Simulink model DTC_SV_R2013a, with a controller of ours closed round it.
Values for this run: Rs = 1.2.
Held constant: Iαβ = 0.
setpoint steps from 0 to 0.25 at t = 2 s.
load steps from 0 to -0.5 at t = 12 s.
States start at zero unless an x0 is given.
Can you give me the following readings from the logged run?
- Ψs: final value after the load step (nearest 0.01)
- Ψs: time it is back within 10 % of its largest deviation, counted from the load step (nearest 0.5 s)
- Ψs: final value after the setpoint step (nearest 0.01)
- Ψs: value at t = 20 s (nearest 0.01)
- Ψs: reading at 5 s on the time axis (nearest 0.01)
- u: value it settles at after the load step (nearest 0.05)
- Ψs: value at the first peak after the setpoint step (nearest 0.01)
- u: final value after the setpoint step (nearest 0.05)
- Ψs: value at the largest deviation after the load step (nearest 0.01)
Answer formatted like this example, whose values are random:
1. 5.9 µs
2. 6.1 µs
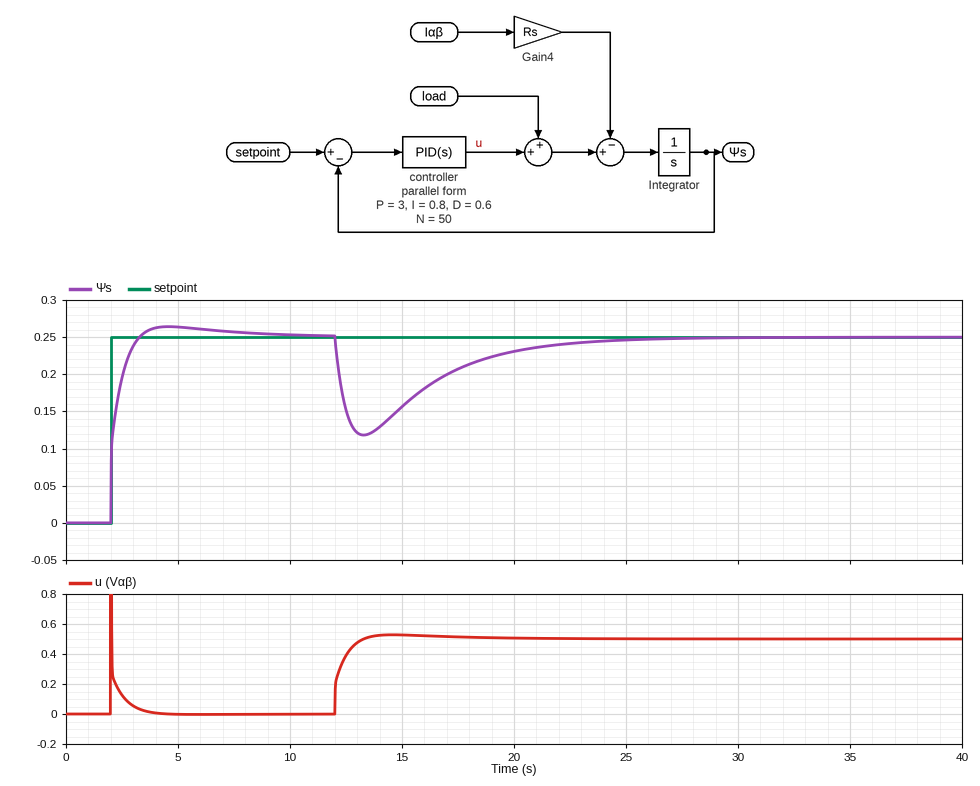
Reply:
1. 0.25
2. 9.0 s
3. 0.25
4. 0.23
5. 0.26
6. 0.50
7. 0.26
8. 0.00
9. 0.12
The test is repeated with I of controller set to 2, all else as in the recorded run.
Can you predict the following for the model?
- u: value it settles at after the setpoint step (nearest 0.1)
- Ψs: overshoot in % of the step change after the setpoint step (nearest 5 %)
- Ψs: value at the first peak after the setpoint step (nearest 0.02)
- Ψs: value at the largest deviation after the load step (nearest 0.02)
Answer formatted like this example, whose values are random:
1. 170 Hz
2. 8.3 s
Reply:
1. 0.0
2. 10 %
3. 0.28
4. 0.14
